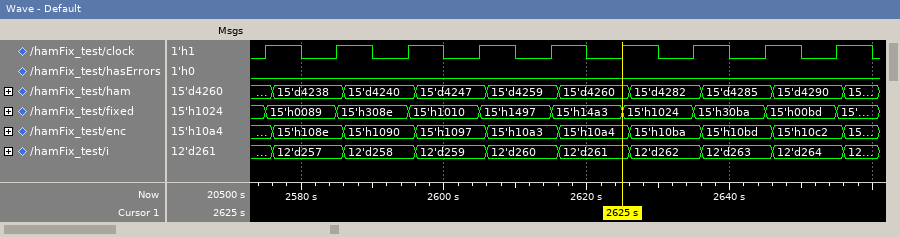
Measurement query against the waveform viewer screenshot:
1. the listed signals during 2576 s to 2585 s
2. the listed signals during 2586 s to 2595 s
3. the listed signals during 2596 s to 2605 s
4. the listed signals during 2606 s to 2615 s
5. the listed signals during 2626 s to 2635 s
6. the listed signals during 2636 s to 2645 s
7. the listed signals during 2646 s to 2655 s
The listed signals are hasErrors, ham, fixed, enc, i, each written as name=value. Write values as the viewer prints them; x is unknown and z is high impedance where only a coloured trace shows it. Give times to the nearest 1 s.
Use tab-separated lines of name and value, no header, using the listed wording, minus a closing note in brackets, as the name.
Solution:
the listed signals during 2576 s to 2585 s	hasErrors=0, ham=15'd4238, fixed=15'h0089, enc=15'h108e, i=12'd257
the listed signals during 2586 s to 2595 s	hasErrors=0, ham=15'd4240, fixed=15'h308e, enc=15'h1090, i=12'd258
the listed signals during 2596 s to 2605 s	hasErrors=0, ham=15'd4247, fixed=15'h1010, enc=15'h1097, i=12'd259
the listed signals during 2606 s to 2615 s	hasErrors=0, ham=15'd4259, fixed=15'h1497, enc=15'h10a3, i=12'd260
the listed signals during 2626 s to 2635 s	hasErrors=0, ham=15'd4282, fixed=15'h1024, enc=15'h10ba, i=12'd262
the listed signals during 2636 s to 2645 s	hasErrors=0, ham=15'd4285, fixed=15'h30ba, enc=15'h10bd, i=12'd263
the listed signals during 2646 s to 2655 s	hasErrors=0, ham=15'd4290, fixed=15'h00bd, enc=15'h10c2, i=12'd264
